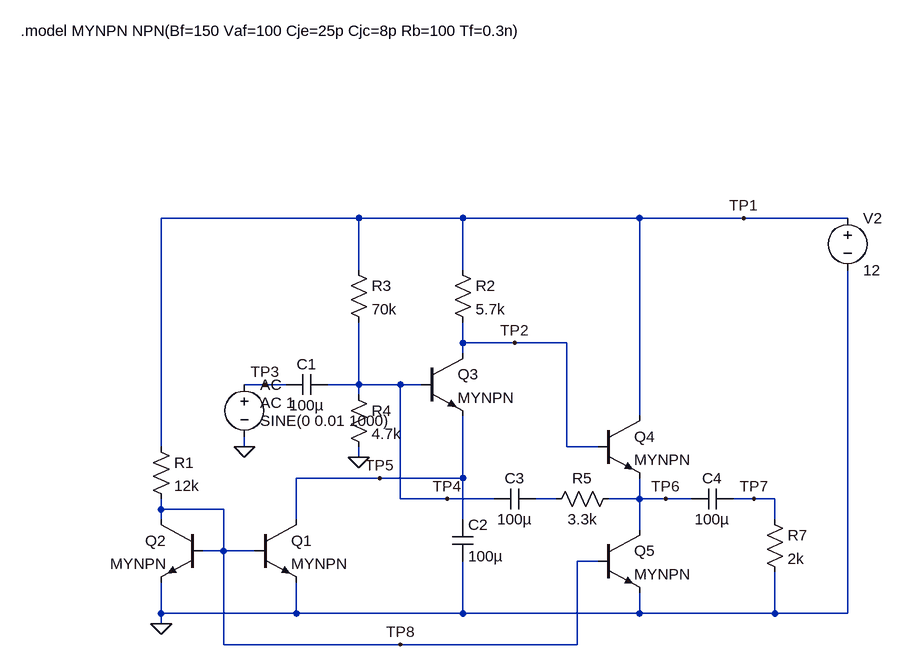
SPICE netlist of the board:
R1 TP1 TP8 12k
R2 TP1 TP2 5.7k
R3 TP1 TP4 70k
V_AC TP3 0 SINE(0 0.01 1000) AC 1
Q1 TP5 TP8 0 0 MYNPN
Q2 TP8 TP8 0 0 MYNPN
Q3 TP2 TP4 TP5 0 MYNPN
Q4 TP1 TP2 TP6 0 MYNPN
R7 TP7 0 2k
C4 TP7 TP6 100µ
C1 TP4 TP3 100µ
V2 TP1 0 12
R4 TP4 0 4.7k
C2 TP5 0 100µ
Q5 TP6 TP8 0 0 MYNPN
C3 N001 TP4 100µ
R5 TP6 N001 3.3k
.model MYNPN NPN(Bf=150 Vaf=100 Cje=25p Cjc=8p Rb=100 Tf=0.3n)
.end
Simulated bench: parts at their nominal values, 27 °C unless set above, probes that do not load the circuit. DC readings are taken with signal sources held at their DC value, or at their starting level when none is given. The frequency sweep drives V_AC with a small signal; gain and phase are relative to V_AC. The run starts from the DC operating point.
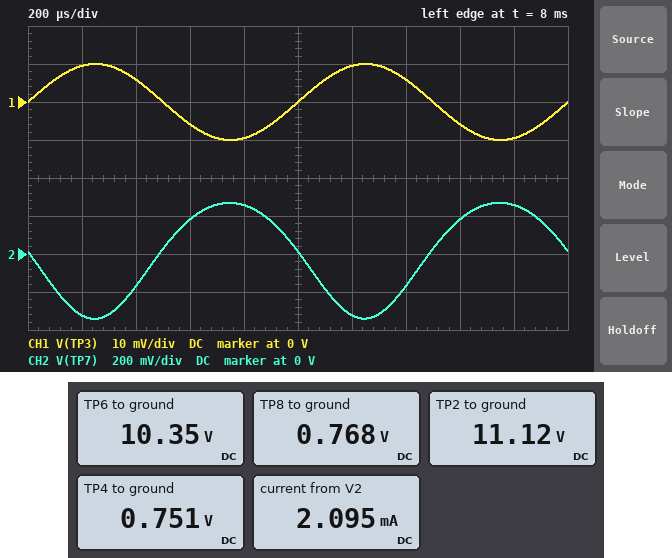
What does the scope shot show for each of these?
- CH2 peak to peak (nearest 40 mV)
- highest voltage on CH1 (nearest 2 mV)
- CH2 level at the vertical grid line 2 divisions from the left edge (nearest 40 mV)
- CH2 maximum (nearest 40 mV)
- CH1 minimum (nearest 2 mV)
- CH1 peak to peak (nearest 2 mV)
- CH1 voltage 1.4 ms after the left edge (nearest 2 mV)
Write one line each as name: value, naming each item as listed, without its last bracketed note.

CH2 peak to peak: 600 mV
highest voltage on CH1: 10 mV
CH2 level at the vertical grid line 2 divisions from the left edge: -160 mV
CH2 maximum: 280 mV
CH1 minimum: -10 mV
CH1 peak to peak: 20 mV
CH1 voltage 1.4 ms after the left edge: 6 mV
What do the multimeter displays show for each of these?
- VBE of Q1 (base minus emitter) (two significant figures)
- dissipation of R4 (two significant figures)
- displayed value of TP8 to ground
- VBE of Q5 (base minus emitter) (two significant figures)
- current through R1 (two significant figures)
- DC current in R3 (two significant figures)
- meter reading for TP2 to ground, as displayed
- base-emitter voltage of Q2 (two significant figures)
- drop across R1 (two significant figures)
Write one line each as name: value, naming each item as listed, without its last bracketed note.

VBE of Q1 (base minus emitter): 770 mV
dissipation of R4: 120 µW
displayed value of TP8 to ground: 0.768 V
VBE of Q5 (base minus emitter): 770 mV
current through R1: 940 µA
DC current in R3: 160 µA
meter reading for TP2 to ground, as displayed: 11.12 V
base-emitter voltage of Q2: 770 mV
drop across R1: 11 V
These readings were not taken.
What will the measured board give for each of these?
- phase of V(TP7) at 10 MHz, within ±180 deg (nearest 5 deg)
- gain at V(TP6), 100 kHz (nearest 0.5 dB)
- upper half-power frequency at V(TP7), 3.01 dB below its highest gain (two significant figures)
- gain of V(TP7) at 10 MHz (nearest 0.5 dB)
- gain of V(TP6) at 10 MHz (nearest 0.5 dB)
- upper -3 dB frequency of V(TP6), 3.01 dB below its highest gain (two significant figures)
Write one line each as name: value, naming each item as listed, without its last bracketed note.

phase of V(TP7) at 10 MHz, within ±180 deg: 80 deg
gain at V(TP6), 100 kHz: 29.5 dB
upper half-power frequency at V(TP7), 3.01 dB below its highest gain: 2.3 MHz
gain of V(TP7) at 10 MHz: 16.0 dB
gain of V(TP6) at 10 MHz: 16.0 dB
upper -3 dB frequency of V(TP6), 3.01 dB below its highest gain: 2.3 MHz
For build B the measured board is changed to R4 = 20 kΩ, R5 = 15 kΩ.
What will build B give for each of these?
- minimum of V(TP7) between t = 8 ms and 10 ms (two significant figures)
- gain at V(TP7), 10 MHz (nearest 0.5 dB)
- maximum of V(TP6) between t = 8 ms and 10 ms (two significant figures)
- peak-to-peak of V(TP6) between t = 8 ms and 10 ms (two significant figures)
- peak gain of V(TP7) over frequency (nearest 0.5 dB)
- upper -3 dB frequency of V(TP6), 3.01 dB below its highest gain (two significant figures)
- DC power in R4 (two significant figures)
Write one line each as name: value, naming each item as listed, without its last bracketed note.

minimum of V(TP7) between t = 8 ms and 10 ms: -1.7 V
gain at V(TP7), 10 MHz: 26.5 dB
maximum of V(TP6) between t = 8 ms and 10 ms: 7.6 V
peak-to-peak of V(TP6) between t = 8 ms and 10 ms: 3.3 V
peak gain of V(TP7) over frequency: 45.0 dB
upper -3 dB frequency of V(TP6), 3.01 dB below its highest gain: 1.2 MHz
DC power in R4: 330 µW
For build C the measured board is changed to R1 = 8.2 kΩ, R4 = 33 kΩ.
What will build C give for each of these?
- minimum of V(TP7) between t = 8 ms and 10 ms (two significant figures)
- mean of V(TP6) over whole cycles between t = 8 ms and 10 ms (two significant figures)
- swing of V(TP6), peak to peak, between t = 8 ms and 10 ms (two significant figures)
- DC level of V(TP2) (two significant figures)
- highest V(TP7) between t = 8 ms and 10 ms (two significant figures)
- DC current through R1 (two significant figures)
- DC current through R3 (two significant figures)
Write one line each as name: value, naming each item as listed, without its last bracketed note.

minimum of V(TP7) between t = 8 ms and 10 ms: -1.2 V
mean of V(TP6) over whole cycles between t = 8 ms and 10 ms: 3.5 V
swing of V(TP6), peak to peak, between t = 8 ms and 10 ms: 3.2 V
DC level of V(TP2): 4.2 V
highest V(TP7) between t = 8 ms and 10 ms: 2.0 V
DC current through R1: 1.4 mA
DC current through R3: 120 µA
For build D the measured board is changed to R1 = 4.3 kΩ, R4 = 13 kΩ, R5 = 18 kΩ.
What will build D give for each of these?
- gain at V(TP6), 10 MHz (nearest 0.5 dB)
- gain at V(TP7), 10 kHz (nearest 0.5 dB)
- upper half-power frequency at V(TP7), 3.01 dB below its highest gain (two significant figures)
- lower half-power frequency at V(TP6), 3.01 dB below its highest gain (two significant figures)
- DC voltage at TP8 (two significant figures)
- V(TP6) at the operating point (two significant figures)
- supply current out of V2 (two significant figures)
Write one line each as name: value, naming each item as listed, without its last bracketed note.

gain at V(TP6), 10 MHz: -15.5 dB
gain at V(TP7), 10 kHz: -53.5 dB
upper half-power frequency at V(TP7), 3.01 dB below its highest gain: 68 MHz
lower half-power frequency at V(TP6), 3.01 dB below its highest gain: 12 MHz
DC voltage at TP8: 800 mV
V(TP6) at the operating point: 18 mV
supply current out of V2: 4.8 mA
